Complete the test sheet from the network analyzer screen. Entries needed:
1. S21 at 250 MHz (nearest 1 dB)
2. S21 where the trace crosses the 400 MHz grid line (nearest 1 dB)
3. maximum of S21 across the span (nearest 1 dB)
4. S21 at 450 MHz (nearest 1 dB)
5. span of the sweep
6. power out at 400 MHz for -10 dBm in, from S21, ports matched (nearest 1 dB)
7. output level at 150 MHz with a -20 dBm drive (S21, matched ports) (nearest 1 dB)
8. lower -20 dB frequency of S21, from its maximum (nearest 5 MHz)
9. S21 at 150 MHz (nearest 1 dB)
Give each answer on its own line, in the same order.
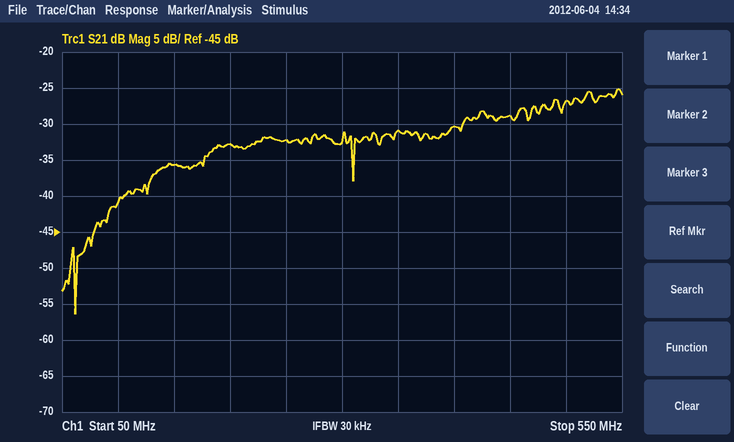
-32 dB
-30 dB
-25 dB
-29 dB
500 MHz
-40 dBm
-56 dBm
80 MHz
-36 dB
